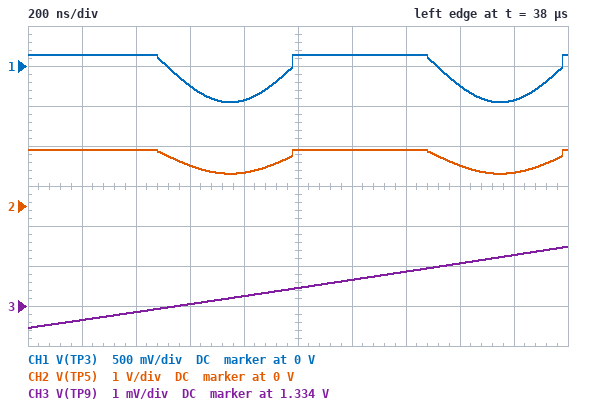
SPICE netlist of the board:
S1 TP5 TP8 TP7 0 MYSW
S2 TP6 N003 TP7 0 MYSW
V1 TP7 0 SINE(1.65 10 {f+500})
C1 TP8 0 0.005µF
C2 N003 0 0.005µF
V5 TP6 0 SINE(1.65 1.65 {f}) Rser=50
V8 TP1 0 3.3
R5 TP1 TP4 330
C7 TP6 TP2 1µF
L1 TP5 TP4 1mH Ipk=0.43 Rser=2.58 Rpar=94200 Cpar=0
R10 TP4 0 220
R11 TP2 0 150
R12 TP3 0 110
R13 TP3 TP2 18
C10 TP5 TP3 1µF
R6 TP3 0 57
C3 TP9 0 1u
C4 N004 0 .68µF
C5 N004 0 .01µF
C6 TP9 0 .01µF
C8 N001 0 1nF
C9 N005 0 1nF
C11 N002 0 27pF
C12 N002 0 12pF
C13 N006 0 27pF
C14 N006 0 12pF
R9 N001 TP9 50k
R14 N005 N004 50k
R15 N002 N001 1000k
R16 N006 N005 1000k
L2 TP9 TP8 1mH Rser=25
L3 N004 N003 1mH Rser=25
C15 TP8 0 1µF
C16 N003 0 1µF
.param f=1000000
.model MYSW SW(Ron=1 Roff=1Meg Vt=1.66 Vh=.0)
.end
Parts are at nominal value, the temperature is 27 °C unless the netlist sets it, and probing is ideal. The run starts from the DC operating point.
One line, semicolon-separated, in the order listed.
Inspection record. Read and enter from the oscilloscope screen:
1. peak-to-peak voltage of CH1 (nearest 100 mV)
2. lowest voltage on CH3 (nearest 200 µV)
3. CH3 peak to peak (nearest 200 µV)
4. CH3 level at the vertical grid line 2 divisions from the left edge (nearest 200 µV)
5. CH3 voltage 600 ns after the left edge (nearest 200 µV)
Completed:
600 mV; 1.3334 V; 2.0 mV; 1.3338 V; 1.3340 V
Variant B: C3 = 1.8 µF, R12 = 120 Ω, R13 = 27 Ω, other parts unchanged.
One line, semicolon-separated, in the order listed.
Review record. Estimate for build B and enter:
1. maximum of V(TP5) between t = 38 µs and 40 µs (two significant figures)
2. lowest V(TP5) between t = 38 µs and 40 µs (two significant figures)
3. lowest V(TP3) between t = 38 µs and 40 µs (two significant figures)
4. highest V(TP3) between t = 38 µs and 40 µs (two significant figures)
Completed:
1.4 V; 850 mV; -420 mV; 120 mV
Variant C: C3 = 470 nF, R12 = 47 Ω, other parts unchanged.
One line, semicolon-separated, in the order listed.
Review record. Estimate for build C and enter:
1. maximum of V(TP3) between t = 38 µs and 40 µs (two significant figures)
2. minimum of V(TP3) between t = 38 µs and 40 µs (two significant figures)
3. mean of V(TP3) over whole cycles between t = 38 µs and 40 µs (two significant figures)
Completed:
130 mV; -360 mV; -43 mV
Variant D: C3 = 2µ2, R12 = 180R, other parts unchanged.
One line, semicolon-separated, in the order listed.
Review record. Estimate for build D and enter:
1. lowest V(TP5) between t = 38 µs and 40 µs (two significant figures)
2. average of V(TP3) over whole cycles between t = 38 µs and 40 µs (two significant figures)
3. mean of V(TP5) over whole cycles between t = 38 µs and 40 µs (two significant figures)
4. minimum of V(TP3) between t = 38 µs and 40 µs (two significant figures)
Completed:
770 mV; -75 mV; 1.2 V; -490 mV
